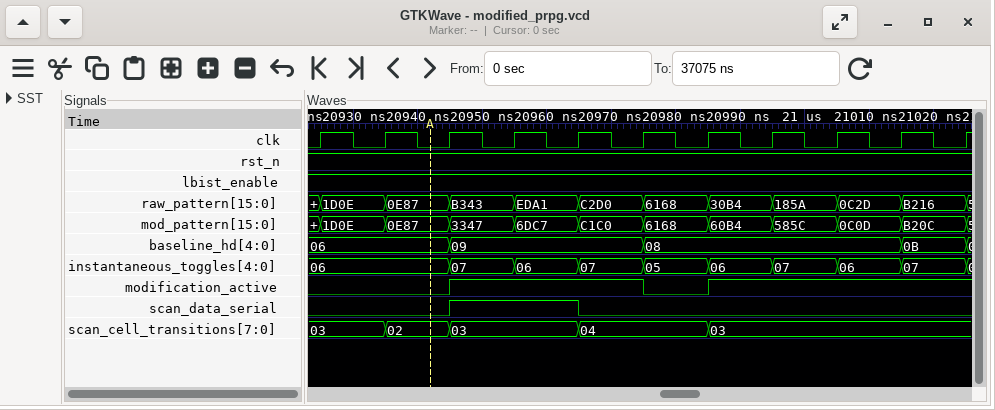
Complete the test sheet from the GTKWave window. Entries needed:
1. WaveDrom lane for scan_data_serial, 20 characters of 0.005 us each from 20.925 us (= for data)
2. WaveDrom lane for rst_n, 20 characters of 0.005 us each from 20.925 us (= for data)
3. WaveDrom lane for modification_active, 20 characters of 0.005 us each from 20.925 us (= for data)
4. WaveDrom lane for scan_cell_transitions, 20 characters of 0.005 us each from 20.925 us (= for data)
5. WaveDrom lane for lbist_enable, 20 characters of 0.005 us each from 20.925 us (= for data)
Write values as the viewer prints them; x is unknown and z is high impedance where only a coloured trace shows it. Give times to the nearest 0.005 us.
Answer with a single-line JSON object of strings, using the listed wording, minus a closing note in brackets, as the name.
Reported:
{"WaveDrom lane for scan_data_serial, 20 characters of 0.005 us each from 20.925 us": "{name: 'scan_data_serial', wave: '0...1...0...........'}", "WaveDrom lane for rst_n, 20 characters of 0.005 us each from 20.925 us": "{name: 'rst_n', wave: '1...................'}", "WaveDrom lane for modification_active, 20 characters of 0.005 us each from 20.925 us": "{name: 'modification_active', wave: '0...1.....0.1.......'}", "WaveDrom lane for scan_cell_transitions, 20 characters of 0.005 us each from 20.925 us": "{name: 'scan_cell_transitions', wave: '=.=.=...=...=.......', data: '03 02 03 04 03'}", "WaveDrom lane for lbist_enable, 20 characters of 0.005 us each from 20.925 us": "{name: 'lbist_enable', wave: '1...................'}"}
